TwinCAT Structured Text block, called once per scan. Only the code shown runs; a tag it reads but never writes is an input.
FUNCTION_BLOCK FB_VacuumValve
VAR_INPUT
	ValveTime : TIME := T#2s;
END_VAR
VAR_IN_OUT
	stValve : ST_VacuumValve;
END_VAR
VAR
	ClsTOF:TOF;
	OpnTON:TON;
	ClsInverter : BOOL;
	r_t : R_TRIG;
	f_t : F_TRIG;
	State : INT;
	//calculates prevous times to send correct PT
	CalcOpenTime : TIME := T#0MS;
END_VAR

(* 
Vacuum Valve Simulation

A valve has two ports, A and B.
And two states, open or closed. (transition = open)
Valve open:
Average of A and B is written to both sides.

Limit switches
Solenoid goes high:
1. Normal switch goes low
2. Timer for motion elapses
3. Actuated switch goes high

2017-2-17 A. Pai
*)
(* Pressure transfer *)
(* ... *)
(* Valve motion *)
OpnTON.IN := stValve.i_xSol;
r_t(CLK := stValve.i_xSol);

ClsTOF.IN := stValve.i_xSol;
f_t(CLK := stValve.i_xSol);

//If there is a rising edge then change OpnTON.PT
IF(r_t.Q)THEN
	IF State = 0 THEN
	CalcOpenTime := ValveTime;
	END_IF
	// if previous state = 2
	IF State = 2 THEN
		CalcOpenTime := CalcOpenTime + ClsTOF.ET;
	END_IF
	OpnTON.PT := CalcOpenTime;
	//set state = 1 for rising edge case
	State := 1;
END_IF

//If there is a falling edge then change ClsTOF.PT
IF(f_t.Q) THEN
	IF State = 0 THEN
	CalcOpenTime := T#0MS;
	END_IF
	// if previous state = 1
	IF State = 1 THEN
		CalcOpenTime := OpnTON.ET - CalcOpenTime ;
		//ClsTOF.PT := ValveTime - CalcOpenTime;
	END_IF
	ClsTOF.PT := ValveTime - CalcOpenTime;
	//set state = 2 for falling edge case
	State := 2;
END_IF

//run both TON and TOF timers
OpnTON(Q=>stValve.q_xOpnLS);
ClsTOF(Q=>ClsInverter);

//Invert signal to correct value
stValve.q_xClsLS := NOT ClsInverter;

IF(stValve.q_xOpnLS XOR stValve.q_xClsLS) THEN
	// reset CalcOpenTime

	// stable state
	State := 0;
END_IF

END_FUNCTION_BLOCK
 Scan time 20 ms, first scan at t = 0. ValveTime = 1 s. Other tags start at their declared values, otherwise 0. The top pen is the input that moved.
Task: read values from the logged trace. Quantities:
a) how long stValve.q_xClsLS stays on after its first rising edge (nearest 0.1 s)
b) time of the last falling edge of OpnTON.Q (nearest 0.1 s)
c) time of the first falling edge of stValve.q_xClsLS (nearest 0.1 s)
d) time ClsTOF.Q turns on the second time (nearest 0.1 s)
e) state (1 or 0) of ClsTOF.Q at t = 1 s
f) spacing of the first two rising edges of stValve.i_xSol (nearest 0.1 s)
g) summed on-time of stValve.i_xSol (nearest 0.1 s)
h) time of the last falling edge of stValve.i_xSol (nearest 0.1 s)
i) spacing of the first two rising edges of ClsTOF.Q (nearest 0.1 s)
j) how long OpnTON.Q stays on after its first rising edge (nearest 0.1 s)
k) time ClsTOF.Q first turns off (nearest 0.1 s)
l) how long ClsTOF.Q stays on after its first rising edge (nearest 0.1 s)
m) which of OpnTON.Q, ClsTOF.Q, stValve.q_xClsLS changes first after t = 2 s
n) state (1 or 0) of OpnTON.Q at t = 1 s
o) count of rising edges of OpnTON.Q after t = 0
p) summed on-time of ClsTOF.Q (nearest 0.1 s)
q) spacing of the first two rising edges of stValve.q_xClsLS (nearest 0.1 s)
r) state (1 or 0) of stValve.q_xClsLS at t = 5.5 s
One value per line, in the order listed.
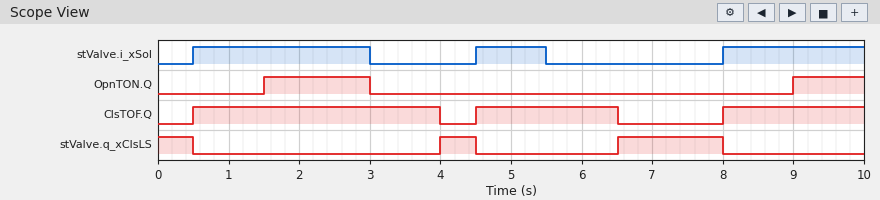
0.5 s
3.0 s
0.5 s
4.5 s
1
4.0 s
5.5 s
5.5 s
4.0 s
1.5 s
4.0 s
3.5 s
OpnTON.Q
0
2
7.5 s
2.5 s
0
